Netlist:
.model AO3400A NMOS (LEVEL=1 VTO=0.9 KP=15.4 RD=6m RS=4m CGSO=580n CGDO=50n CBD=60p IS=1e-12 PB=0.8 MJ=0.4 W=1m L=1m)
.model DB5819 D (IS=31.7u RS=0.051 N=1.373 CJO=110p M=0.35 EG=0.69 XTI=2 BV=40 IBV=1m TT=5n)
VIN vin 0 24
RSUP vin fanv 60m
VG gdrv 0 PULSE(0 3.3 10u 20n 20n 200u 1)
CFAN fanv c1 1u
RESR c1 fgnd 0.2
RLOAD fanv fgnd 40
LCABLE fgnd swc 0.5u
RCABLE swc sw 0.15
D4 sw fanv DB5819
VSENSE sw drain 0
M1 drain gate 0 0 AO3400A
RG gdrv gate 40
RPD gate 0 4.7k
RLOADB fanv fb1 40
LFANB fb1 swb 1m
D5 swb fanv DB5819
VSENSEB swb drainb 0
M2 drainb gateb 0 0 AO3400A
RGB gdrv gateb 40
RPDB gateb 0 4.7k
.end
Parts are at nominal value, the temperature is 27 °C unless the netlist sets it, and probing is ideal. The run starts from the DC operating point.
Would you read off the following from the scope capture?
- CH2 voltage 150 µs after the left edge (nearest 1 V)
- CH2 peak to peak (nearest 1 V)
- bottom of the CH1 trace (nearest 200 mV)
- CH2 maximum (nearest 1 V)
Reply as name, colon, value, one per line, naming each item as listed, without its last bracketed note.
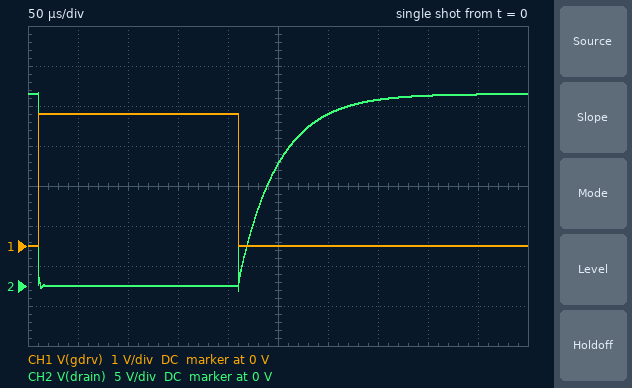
CH2 voltage 150 µs after the left edge: 0 V
CH2 peak to peak: 25 V
bottom of the CH1 trace: 0 V
CH2 maximum: 24 V
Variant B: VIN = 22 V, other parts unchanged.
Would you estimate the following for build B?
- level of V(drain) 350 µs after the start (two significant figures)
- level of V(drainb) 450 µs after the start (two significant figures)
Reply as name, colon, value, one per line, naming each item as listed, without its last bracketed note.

level of V(drain) 350 µs after the start: 21 V
level of V(drainb) 450 µs after the start: 22 V
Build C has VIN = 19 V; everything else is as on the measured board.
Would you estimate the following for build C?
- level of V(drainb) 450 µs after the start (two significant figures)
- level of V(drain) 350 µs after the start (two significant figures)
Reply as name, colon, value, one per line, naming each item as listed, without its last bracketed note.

level of V(drainb) 450 µs after the start: 19 V
level of V(drain) 350 µs after the start: 18 V
